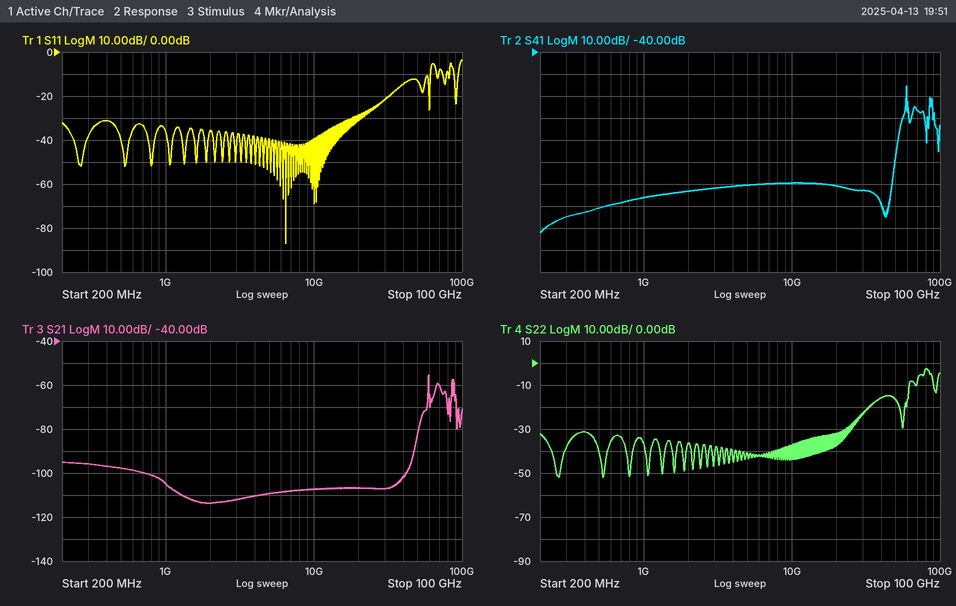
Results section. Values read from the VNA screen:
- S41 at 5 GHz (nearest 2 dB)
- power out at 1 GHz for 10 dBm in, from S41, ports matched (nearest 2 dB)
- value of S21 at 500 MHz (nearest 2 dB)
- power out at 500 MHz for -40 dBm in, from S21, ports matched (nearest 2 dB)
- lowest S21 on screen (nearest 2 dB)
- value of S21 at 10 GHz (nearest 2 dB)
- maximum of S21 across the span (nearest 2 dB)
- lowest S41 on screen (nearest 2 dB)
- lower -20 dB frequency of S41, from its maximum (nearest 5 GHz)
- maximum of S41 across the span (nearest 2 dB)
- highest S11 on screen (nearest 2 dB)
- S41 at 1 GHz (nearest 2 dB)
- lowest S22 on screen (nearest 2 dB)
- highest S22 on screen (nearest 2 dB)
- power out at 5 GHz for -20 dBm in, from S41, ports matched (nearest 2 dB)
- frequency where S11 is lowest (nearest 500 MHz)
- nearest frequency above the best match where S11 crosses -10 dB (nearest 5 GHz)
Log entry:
-100 dB
-96 dBm
-98 dB
-138 dBm
-114 dB
-108 dB
-56 dB
-122 dB
55 GHz
-56 dB
-4 dB
-106 dB
-52 dB
-2 dB
-120 dBm
6.5 GHz
60 GHz
